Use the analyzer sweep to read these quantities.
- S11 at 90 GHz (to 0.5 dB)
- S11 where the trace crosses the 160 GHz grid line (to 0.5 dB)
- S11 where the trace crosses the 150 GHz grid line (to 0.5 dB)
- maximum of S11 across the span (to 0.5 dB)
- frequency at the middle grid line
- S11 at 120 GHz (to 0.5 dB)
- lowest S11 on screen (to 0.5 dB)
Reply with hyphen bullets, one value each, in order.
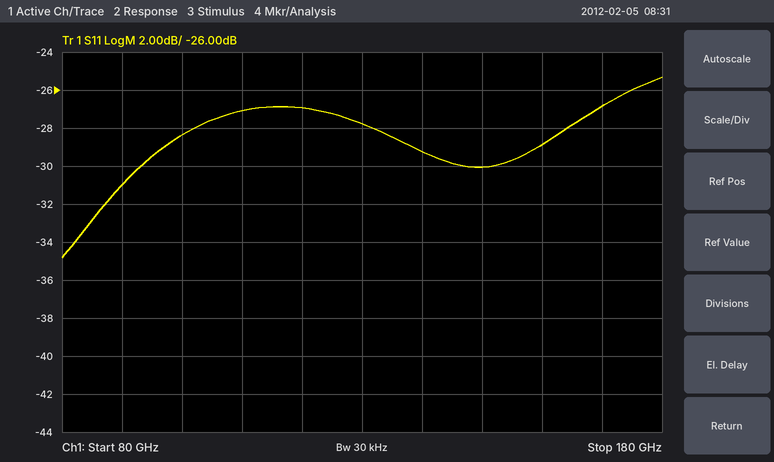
- -31.0 dB
- -29.0 dB
- -30.0 dB
- -25.5 dB
- 130 GHz
- -27.0 dB
- -35.0 dB
